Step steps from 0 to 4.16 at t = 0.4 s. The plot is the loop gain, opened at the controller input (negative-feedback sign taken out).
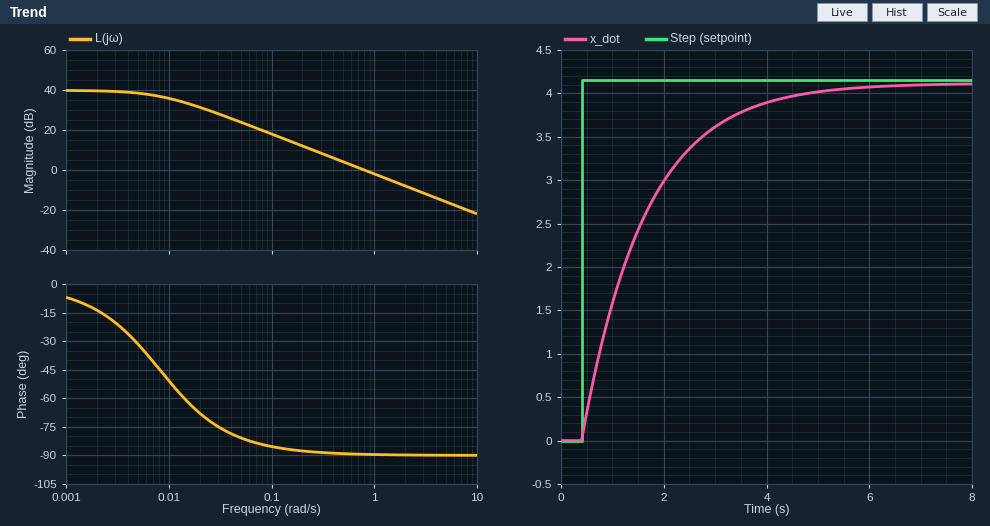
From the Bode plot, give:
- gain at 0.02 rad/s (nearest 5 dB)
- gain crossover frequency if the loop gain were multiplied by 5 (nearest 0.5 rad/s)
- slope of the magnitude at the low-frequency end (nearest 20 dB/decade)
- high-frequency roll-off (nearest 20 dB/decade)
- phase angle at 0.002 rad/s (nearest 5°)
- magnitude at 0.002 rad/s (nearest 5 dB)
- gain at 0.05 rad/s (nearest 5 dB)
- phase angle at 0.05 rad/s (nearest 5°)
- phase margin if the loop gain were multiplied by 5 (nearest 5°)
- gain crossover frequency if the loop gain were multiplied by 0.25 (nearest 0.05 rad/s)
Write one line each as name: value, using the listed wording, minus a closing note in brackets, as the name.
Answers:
gain at 0.02 rad/s: 30 dB
gain crossover frequency if the loop gain were multiplied by 5: 4.0 rad/s
slope of the magnitude at the low-frequency end: 0 dB/decade
high-frequency roll-off: -20 dB/decade
phase angle at 0.002 rad/s: -15°
magnitude at 0.002 rad/s: 40 dB
gain at 0.05 rad/s: 25 dB
phase angle at 0.05 rad/s: -80°
phase margin if the loop gain were multiplied by 5: 90°
gain crossover frequency if the loop gain were multiplied by 0.25: 0.20 rad/s
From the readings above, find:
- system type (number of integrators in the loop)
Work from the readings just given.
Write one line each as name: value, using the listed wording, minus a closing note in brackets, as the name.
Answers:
system type: 0
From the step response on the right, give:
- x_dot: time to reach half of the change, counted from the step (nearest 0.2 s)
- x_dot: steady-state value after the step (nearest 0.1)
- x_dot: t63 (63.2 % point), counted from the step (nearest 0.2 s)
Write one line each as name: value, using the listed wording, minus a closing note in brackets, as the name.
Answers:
x_dot: time to reach half of the change, counted from the step: 0.8 s
x_dot: steady-state value after the step: 4.1
x_dot: t63 (63.2 % point), counted from the step: 1.2 s
